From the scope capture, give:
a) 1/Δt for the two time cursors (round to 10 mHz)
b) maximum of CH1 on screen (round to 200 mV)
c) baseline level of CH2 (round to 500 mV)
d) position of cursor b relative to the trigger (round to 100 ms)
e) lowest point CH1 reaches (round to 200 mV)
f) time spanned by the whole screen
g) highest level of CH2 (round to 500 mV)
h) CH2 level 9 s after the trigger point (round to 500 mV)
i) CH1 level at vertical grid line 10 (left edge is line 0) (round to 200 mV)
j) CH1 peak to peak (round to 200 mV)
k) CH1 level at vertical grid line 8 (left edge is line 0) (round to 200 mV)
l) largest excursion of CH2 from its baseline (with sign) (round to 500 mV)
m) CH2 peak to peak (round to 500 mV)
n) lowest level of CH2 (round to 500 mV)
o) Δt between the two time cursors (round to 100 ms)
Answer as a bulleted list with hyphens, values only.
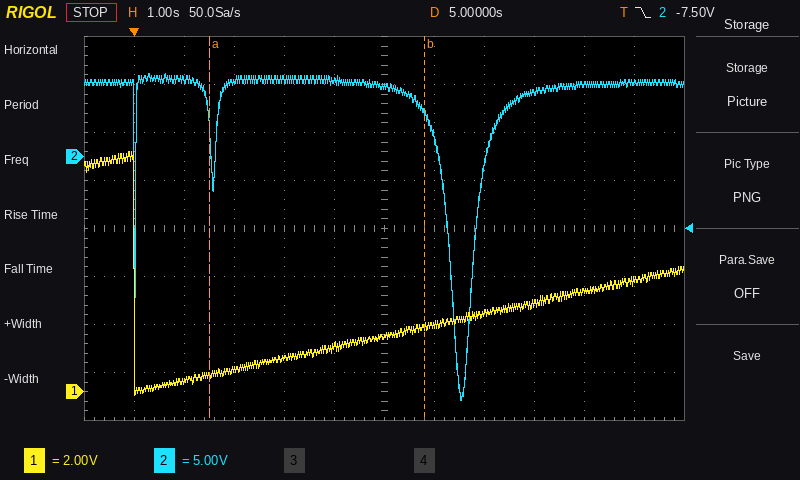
- 230 mHz
- 10.0 V
- 7.5 V
- +5.8 s
- -200 mV
- 12 s
- 8.5 V
- 7.5 V
- 4.2 V
- 10.2 V
- 3.2 V
- -33.0 V
- 34.0 V
- -25.5 V
- 4.3 s
